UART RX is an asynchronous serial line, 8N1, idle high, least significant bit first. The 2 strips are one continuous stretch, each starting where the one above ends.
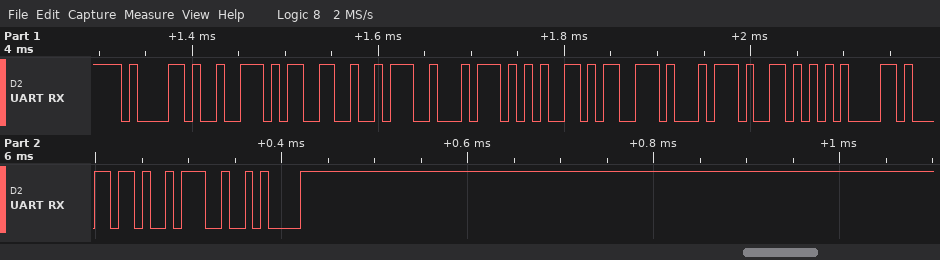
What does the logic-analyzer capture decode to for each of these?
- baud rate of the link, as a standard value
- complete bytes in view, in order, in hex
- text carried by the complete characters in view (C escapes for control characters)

115200 baud
0x61 0x72 0x33 0x3A 0x74 0x65 0x73 0x74 0x56 0x61 0x6C 0x3A 0x0A
"ar3:testVal:\n"
